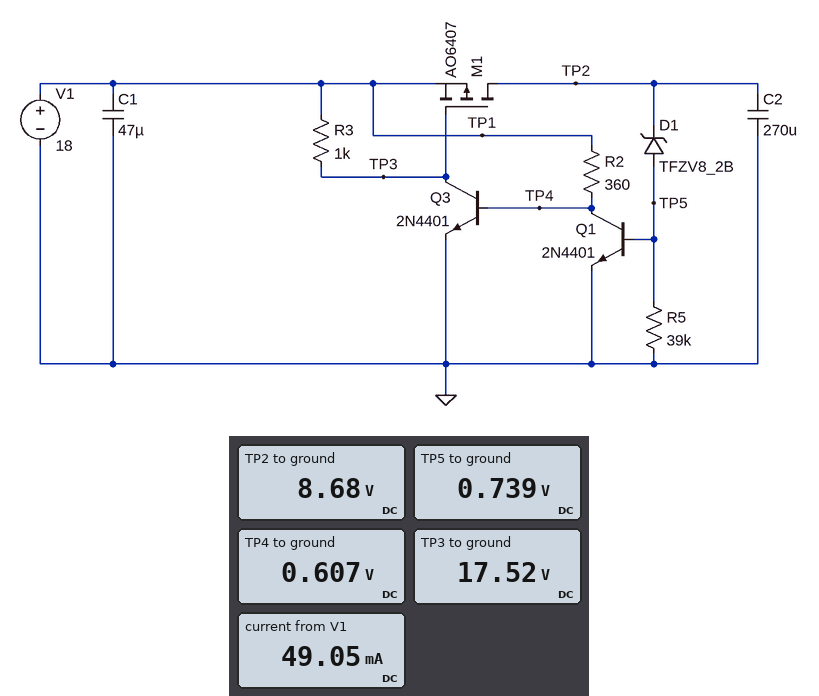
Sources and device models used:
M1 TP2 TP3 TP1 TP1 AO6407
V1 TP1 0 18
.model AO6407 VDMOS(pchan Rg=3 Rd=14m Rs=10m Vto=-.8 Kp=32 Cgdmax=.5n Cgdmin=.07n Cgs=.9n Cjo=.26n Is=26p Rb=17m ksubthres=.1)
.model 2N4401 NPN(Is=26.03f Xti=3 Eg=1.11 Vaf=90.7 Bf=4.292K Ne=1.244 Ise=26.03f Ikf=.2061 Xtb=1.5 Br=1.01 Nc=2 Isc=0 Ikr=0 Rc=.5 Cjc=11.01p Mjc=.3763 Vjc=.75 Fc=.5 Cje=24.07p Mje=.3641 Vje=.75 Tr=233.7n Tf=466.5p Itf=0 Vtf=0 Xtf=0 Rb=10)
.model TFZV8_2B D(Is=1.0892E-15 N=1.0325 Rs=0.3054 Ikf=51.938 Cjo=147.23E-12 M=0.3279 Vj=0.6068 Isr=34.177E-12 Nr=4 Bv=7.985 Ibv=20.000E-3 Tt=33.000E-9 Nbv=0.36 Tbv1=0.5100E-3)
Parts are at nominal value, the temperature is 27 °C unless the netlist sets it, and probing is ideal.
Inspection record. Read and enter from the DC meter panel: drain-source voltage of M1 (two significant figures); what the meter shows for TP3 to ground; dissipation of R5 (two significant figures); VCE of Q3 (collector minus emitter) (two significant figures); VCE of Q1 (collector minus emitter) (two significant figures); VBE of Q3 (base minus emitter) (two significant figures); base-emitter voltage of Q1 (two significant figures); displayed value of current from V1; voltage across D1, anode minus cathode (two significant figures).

-9.3 V
17.52 V
14 µW
18 V
610 mV
610 mV
740 mV
49.05 mA
-7.9 V
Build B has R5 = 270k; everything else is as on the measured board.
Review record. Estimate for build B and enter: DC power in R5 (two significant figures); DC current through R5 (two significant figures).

2.0 µW
2.7 µA
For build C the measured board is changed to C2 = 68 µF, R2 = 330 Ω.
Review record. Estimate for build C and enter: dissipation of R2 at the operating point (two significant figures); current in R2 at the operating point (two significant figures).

920 mW
53 mA
